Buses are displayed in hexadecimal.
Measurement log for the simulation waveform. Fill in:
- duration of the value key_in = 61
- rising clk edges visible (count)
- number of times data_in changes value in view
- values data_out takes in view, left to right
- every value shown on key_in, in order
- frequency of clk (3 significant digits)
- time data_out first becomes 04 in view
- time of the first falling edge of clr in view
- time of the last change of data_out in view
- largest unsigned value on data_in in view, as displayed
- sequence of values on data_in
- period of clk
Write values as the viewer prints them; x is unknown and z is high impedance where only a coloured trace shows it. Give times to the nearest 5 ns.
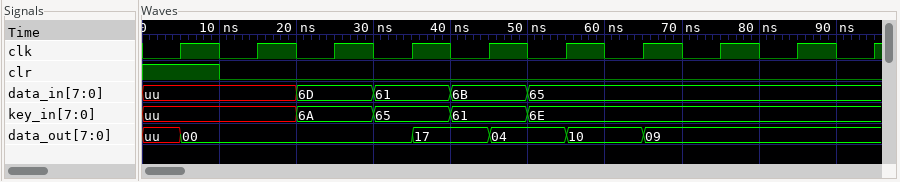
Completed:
10 ns
10
4
uu, 00, 17, 04, 10, 09
uu, 6A, 65, 61, 6E
100 MHz
45 ns
10 ns
65 ns
6D
uu, 6D, 61, 6B, 65
10 ns
